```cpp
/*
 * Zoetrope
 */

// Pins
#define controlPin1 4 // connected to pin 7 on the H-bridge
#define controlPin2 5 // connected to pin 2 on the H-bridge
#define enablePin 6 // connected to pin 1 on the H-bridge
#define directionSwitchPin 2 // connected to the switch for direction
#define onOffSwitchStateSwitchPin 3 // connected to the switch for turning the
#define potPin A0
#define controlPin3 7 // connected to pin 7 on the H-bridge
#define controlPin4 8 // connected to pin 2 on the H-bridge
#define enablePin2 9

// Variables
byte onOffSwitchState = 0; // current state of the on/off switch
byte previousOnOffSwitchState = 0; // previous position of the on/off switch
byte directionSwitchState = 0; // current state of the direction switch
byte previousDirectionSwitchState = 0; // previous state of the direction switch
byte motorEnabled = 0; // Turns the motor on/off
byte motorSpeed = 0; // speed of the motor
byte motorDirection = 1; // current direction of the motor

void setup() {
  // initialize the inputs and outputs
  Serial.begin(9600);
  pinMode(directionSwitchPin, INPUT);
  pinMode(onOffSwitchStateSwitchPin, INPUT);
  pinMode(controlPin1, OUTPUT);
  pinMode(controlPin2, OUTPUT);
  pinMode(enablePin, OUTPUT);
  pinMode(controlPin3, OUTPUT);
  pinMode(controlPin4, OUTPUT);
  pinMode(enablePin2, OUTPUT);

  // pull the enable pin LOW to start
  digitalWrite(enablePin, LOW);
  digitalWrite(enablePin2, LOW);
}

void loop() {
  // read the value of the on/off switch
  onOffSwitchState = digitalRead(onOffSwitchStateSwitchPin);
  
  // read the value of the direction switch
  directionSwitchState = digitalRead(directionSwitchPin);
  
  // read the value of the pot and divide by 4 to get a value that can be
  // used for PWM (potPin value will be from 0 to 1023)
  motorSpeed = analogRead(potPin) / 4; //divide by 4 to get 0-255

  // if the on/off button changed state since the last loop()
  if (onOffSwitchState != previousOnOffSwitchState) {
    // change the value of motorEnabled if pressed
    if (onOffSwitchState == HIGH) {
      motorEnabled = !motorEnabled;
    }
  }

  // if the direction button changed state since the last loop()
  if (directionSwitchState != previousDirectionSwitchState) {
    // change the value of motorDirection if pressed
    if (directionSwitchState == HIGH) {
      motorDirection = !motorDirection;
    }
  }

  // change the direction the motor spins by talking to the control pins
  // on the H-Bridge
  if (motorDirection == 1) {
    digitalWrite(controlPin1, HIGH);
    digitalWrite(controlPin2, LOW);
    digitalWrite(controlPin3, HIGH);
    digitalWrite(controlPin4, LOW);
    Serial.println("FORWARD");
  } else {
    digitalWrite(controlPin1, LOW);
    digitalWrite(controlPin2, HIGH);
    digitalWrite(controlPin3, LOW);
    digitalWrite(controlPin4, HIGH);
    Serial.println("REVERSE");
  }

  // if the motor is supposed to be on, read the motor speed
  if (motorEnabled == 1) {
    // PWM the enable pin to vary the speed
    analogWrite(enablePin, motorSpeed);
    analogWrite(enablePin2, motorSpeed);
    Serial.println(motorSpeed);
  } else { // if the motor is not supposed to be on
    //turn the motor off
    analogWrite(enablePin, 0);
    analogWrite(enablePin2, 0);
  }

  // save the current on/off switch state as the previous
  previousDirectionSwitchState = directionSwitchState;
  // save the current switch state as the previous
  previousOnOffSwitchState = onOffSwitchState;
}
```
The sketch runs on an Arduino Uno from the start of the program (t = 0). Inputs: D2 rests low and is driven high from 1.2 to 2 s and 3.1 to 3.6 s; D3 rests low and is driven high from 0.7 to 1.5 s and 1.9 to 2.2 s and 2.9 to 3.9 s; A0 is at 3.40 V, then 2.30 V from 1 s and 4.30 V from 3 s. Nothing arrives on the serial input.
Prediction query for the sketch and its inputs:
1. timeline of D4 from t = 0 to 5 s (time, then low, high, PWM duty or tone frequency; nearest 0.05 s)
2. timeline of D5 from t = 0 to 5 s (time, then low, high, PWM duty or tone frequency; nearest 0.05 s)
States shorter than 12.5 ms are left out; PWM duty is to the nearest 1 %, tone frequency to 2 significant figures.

0 s high; 1.2 s low; 3.1 s high
0 s low; 1.2 s high; 3.1 s low
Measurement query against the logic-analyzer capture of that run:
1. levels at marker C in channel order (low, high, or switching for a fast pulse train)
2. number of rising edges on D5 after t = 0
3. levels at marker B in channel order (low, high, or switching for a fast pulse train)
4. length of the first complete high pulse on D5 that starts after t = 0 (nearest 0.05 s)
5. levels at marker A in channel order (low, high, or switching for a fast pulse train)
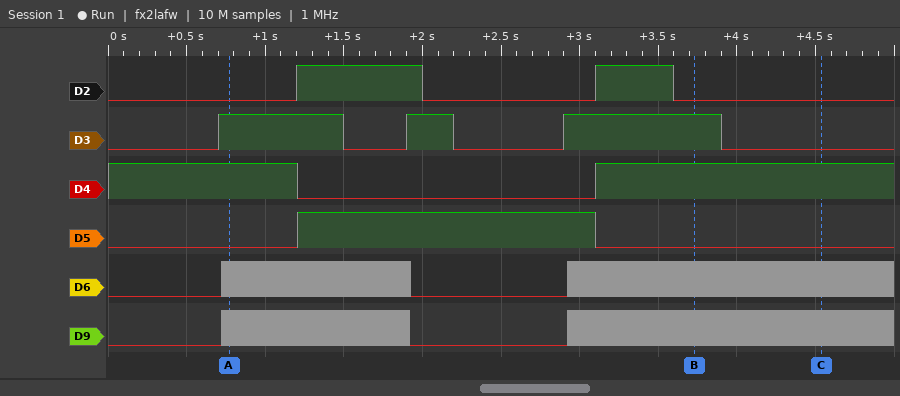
D2 low, D3 low, D4 high, D5 low, D6 switching, D9 switching
1
D2 low, D3 high, D4 high, D5 low, D6 switching, D9 switching
1.90 s
D2 low, D3 high, D4 high, D5 low, D6 switching, D9 switching
